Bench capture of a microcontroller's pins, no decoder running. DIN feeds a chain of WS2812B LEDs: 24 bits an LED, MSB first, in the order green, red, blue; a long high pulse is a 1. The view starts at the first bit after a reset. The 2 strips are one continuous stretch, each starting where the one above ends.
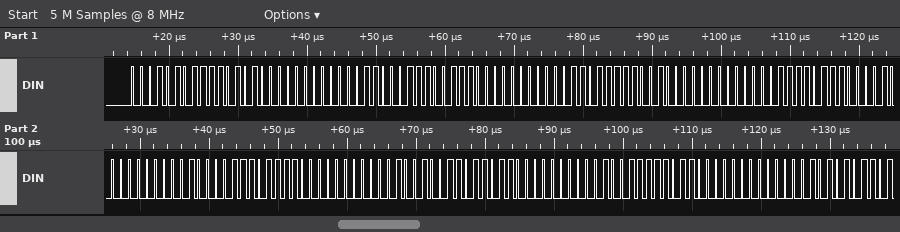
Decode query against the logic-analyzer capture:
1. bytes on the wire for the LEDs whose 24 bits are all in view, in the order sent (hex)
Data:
15 EA 00 18 E7 00 1B E4 00 1E E1 00 21 DE 00 24 DB 00 27 D8 00
